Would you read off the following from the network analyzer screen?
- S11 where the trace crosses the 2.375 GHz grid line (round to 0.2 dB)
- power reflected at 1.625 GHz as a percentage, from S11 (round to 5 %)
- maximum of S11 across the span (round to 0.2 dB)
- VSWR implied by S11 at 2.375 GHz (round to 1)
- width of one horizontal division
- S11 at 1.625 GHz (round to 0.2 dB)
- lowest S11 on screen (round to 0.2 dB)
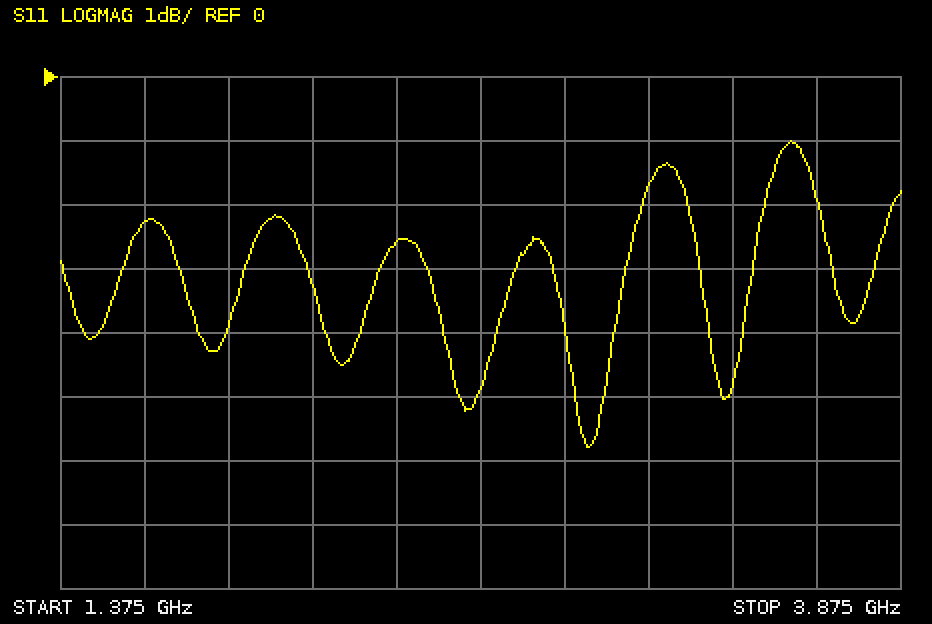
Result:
-2.6 dB
60 %
-1.0 dB
7
250 MHz
-2.2 dB
-5.8 dB
